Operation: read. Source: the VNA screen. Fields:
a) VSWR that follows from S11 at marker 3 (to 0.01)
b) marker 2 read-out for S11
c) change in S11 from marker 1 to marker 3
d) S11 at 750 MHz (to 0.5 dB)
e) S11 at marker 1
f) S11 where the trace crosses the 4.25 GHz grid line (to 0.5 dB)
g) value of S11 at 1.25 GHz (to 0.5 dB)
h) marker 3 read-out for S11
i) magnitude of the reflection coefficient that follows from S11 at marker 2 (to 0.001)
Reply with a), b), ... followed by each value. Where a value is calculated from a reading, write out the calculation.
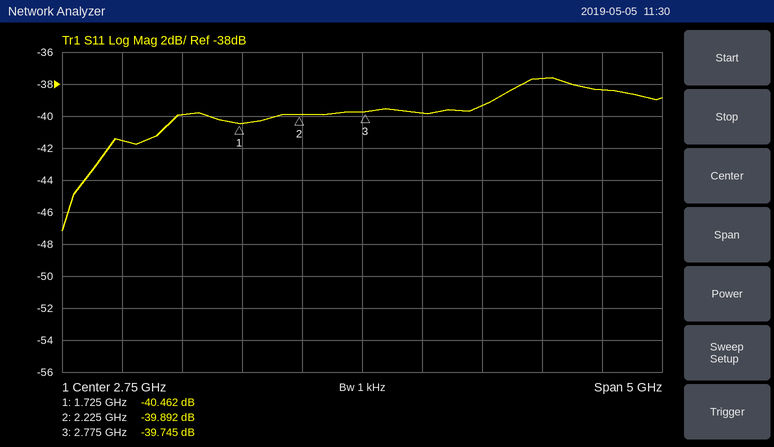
a) (1 + 0.0103)/(1 − 0.0103) ≈ 1.02
b) -39.892 dB
c) -39.745 − (-40.462) = 0.717 dB
d) -41.5 dB
e) -40.462 dB
f) -37.5 dB
g) -40.0 dB
h) -39.745 dB
i) 10^(-39.892/20) ≈ 0.010
